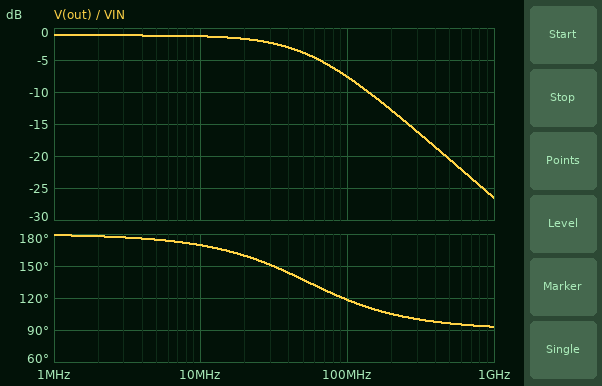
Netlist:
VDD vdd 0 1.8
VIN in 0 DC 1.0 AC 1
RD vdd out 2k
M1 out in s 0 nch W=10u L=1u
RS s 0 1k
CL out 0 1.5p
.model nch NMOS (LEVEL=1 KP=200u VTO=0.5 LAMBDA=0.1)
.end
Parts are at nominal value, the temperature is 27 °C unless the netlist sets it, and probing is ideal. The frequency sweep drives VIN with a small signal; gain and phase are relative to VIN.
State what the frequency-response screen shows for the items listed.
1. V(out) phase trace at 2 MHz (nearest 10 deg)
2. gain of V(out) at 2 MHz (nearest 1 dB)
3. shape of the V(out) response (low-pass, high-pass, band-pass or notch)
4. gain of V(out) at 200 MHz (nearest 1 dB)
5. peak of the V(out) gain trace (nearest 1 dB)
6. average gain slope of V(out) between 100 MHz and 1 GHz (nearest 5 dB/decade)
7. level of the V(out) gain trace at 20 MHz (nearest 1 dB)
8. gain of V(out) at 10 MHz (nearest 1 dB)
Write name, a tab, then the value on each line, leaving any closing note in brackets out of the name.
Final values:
V(out) phase trace at 2 MHz	180 deg
gain of V(out) at 2 MHz	-1 dB
shape of the V(out) response	low-pass
gain of V(out) at 200 MHz	-13 dB
peak of the V(out) gain trace	-1 dB
average gain slope of V(out) between 100 MHz and 1 GHz	-20 dB/decade
level of the V(out) gain trace at 20 MHz	-2 dB
gain of V(out) at 10 MHz	-1 dB
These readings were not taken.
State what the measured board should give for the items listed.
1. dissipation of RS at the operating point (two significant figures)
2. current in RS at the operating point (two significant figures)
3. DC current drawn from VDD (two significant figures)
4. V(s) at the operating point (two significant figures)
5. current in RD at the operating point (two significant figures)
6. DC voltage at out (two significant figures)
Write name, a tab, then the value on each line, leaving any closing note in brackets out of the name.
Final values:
dissipation of RS at the operating point	21 µW
current in RS at the operating point	140 µA
DC current drawn from VDD	140 µA
V(s) at the operating point	140 mV
current in RD at the operating point	140 µA
DC voltage at out	1.5 V
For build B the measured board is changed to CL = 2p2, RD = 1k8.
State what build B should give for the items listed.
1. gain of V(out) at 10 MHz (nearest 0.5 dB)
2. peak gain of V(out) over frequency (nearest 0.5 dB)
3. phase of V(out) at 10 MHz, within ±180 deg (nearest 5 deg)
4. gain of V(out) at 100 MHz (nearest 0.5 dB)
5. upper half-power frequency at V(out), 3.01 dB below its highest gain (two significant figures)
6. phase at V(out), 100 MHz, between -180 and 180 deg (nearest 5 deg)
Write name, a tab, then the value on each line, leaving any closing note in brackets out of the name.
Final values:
gain of V(out) at 10 MHz	-2.5 dB
peak gain of V(out) over frequency	-2.0 dB
phase of V(out) at 10 MHz, within ±180 deg	165 deg
gain of V(out) at 100 MHz	-10.5 dB
upper half-power frequency at V(out), 3.01 dB below its highest gain	41 MHz
phase at V(out), 100 MHz, between -180 and 180 deg	110 deg
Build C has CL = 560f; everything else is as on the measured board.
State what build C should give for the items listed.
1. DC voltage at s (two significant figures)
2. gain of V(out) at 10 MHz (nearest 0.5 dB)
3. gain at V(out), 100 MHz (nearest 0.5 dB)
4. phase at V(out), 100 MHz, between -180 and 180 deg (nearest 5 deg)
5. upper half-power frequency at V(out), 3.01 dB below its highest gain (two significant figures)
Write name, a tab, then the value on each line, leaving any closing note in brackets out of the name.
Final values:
DC voltage at s	140 mV
gain of V(out) at 10 MHz	-1.0 dB
gain at V(out), 100 MHz	-3.0 dB
phase at V(out), 100 MHz, between -180 and 180 deg	145 deg
upper half-power frequency at V(out), 3.01 dB below its highest gain	140 MHz
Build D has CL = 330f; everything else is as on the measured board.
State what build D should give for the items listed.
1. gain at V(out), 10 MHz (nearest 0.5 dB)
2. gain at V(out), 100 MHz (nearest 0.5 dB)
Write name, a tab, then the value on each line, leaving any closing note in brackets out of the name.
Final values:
gain at V(out), 10 MHz	-1.0 dB
gain at V(out), 100 MHz	-2.0 dB
